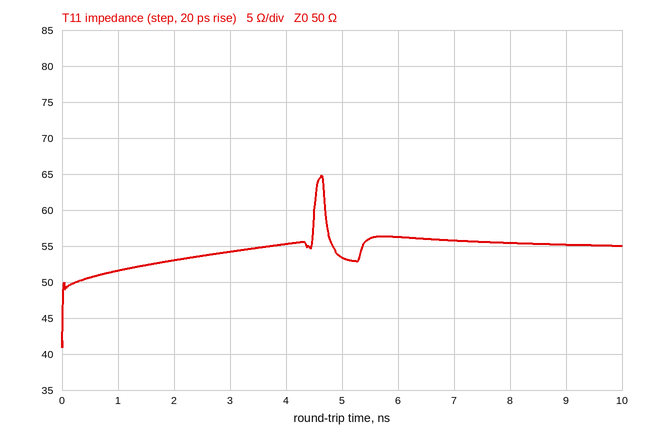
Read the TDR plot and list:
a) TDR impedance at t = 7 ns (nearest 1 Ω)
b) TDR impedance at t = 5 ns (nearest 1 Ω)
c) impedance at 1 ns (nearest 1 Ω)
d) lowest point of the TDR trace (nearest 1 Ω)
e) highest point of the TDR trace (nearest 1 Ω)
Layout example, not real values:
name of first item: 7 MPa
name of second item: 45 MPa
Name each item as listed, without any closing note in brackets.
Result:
TDR impedance at t = 7 ns: 56 Ω
TDR impedance at t = 5 ns: 53 Ω
impedance at 1 ns: 52 Ω
lowest point of the TDR trace: 41 Ω
highest point of the TDR trace: 65 Ω
